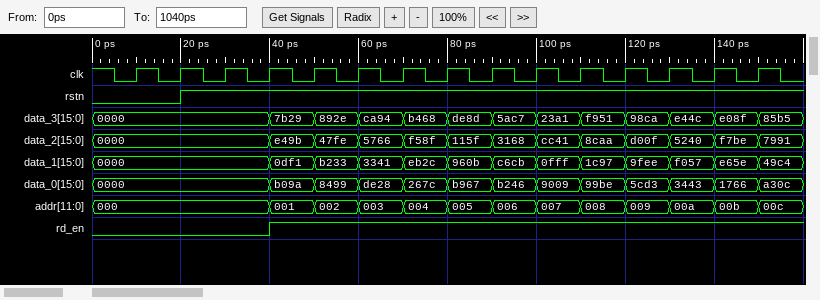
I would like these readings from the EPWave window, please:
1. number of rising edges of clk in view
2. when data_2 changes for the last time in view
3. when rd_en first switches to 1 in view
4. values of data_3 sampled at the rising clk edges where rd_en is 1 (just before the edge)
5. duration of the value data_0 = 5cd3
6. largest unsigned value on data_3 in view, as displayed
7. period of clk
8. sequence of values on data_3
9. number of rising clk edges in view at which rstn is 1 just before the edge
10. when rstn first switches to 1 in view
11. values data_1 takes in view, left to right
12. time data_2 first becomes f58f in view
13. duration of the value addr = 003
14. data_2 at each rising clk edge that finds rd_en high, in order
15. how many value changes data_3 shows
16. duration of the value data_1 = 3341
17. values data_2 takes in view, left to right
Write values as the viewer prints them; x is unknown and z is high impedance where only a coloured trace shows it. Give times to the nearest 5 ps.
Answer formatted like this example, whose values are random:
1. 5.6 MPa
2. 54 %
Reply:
1. 15
2. 150 ps
3. 40 ps
4. 7b29, 892e, ca94, b468, de8d, 5ac7, 23a1, f951, 98ca, e44c, e08f
5. 10 ps
6. f951
7. 10 ps
8. 0000, 7b29, 892e, ca94, b468, de8d, 5ac7, 23a1, f951, 98ca, e44c, e08f, 85b5
9. 13
10. 20 ps
11. 0000, 0df1, b233, 3341, eb2c, 960b, c6cb, 0fff, 1c97, 9fee, f057, e65e, 49c4
12. 70 ps
13. 10 ps
14. e49b, 47fe, 5766, f58f, 115f, 3168, cc41, 8caa, d00f, 5240, f7be
15. 12
16. 10 ps
17. 0000, e49b, 47fe, 5766, f58f, 115f, 3168, cc41, 8caa, d00f, 5240, f7be, 7991
